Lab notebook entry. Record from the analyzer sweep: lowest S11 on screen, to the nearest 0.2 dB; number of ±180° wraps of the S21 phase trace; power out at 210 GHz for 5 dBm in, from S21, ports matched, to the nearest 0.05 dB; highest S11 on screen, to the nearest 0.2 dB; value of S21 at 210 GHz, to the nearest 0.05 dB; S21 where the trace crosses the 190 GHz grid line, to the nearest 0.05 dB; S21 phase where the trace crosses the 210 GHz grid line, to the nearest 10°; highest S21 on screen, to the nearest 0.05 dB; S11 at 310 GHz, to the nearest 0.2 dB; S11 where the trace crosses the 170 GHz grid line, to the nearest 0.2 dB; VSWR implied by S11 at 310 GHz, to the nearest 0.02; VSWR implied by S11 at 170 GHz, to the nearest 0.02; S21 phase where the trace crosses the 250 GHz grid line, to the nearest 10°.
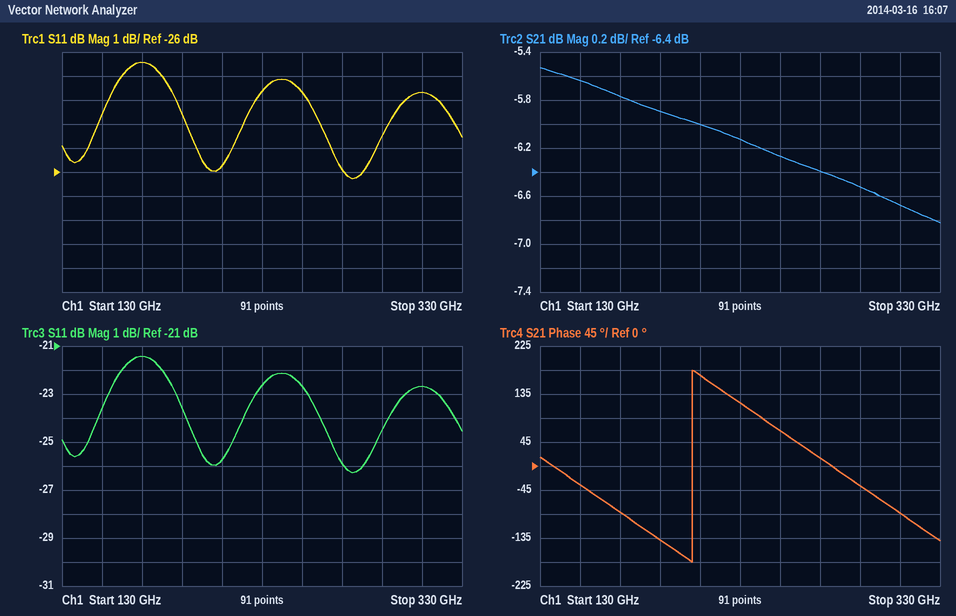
-26.2 dB
1
-1.00 dBm
-21.4 dB
-6.00 dB
-5.90 dB
170°
-5.55 dB
-22.6 dB
-21.4 dB
1.16
1.18
70°
